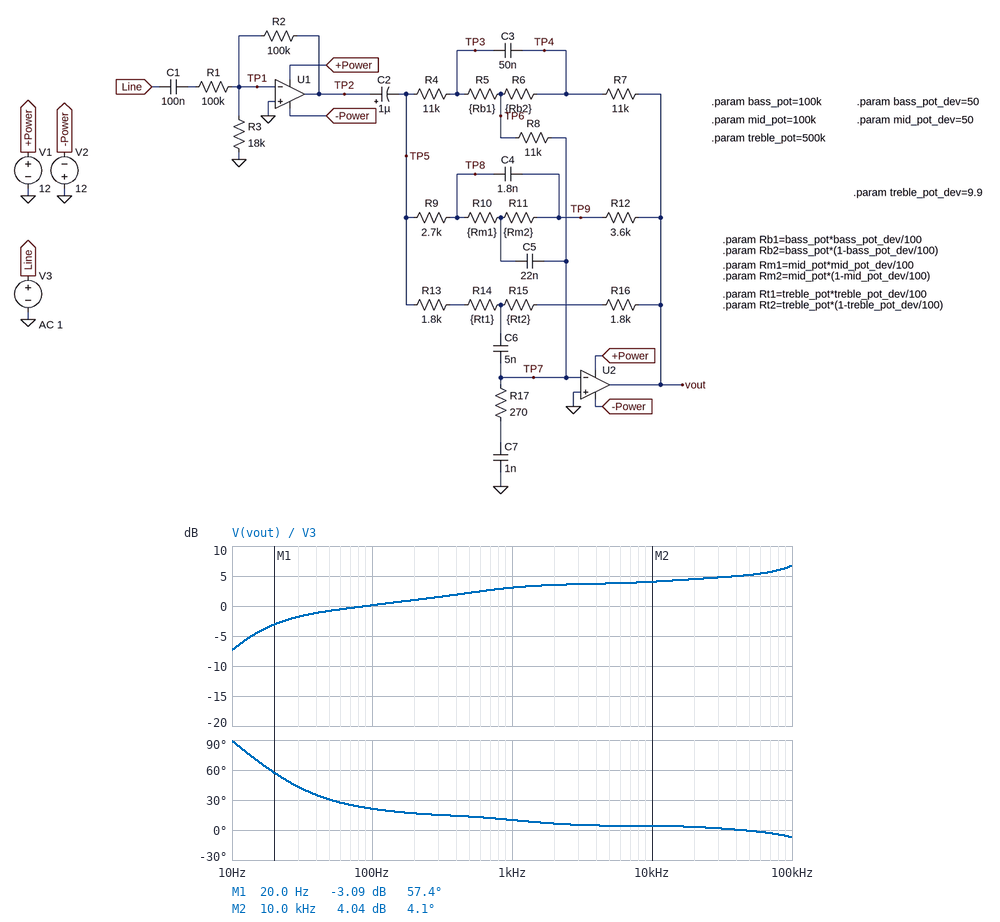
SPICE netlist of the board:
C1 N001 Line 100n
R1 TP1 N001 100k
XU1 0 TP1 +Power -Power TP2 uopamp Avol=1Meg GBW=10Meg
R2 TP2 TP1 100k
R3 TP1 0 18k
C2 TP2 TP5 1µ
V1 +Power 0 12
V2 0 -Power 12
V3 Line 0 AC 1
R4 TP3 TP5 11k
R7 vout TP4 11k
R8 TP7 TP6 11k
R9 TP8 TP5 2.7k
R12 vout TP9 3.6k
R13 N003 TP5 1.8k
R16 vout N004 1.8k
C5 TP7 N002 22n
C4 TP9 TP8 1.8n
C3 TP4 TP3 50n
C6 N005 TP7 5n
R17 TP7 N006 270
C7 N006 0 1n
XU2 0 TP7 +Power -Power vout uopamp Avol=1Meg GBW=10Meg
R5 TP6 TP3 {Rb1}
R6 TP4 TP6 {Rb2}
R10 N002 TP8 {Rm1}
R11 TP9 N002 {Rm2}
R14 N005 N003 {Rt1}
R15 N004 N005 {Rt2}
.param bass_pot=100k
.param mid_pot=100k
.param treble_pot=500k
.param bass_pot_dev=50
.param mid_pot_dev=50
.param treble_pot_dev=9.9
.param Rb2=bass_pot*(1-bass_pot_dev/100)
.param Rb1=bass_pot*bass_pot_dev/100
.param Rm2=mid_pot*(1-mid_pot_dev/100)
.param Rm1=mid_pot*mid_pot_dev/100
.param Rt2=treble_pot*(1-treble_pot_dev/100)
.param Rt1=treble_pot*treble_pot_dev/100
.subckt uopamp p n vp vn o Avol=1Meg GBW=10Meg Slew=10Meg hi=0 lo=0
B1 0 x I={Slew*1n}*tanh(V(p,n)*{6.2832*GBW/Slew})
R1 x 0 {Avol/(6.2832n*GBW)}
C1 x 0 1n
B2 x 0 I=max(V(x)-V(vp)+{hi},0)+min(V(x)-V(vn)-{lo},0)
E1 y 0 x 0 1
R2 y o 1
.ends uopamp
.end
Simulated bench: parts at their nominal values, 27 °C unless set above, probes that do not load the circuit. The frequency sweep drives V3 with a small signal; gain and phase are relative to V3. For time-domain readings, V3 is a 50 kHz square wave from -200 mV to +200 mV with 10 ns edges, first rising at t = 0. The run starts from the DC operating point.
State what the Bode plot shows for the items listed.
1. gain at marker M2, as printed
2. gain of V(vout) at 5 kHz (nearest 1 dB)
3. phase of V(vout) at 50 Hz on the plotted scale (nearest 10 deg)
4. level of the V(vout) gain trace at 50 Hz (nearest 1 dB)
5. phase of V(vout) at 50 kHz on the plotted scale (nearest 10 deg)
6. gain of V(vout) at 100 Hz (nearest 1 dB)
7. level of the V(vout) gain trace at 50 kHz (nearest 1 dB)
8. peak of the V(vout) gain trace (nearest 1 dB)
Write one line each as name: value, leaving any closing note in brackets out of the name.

gain at marker M2, as printed: 4.04 dB
gain of V(vout) at 5 kHz: 4 dB
phase of V(vout) at 50 Hz on the plotted scale: 30 deg
level of the V(vout) gain trace at 50 Hz: -1 dB
phase of V(vout) at 50 kHz on the plotted scale: 0 deg
gain of V(vout) at 100 Hz: 0 dB
level of the V(vout) gain trace at 50 kHz: 5 dB
peak of the V(vout) gain trace: 7 dB
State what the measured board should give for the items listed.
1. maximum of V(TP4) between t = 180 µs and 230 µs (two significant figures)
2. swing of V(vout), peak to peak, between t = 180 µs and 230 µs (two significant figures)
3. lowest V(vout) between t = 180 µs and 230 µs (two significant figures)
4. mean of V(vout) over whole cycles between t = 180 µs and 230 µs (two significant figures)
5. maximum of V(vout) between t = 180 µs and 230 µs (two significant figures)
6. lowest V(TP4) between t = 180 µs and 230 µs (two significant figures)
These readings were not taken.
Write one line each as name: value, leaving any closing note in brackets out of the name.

maximum of V(TP4) between t = 180 µs and 230 µs: 290 mV
swing of V(vout), peak to peak, between t = 180 µs and 230 µs: 1.4 V
lowest V(vout) between t = 180 µs and 230 µs: -470 mV
mean of V(vout) over whole cycles between t = 180 µs and 230 µs: 250 mV
maximum of V(vout) between t = 180 µs and 230 µs: 970 mV
lowest V(TP4) between t = 180 µs and 230 µs: -160 mV
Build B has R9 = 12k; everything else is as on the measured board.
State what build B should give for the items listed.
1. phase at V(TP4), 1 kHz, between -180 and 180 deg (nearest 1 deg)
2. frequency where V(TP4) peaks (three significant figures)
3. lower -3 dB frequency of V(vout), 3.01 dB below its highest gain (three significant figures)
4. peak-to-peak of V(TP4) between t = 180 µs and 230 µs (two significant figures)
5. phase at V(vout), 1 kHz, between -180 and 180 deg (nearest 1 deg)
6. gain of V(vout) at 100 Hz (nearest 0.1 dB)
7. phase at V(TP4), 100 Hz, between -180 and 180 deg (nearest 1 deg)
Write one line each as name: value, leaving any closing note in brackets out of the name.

phase at V(TP4), 1 kHz, between -180 and 180 deg: -32 deg
frequency where V(TP4) peaks: 273 kHz
lower -3 dB frequency of V(vout), 3.01 dB below its highest gain: 168 kHz
peak-to-peak of V(TP4) between t = 180 µs and 230 µs: 280 mV
phase at V(vout), 1 kHz, between -180 and 180 deg: 6 deg
gain of V(vout) at 100 Hz: -0.2 dB
phase at V(TP4), 100 Hz, between -180 and 180 deg: -10 deg
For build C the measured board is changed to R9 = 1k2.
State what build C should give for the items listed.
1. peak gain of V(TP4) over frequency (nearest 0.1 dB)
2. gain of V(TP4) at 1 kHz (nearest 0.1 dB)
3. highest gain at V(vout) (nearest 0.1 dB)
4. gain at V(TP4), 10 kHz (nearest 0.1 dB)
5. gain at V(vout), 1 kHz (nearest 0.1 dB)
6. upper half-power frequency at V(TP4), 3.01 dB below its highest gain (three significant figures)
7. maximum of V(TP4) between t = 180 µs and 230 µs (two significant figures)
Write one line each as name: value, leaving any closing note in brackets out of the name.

peak gain of V(TP4) over frequency: 9.7 dB
gain of V(TP4) at 1 kHz: -12.3 dB
highest gain at V(vout): 17.4 dB
gain at V(TP4), 10 kHz: -9.9 dB
gain at V(vout), 1 kHz: 3.2 dB
upper half-power frequency at V(TP4), 3.01 dB below its highest gain: 229 kHz
maximum of V(TP4) between t = 180 µs and 230 µs: 450 mV
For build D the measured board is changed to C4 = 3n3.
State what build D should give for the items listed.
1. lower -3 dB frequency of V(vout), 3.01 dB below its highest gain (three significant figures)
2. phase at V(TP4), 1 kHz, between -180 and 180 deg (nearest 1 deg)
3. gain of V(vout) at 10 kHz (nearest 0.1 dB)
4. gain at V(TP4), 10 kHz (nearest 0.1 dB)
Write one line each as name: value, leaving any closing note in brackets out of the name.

lower -3 dB frequency of V(vout), 3.01 dB below its highest gain: 155 kHz
phase at V(TP4), 1 kHz, between -180 and 180 deg: -17 deg
gain of V(vout) at 10 kHz: 4.4 dB
gain at V(TP4), 10 kHz: -10.9 dB
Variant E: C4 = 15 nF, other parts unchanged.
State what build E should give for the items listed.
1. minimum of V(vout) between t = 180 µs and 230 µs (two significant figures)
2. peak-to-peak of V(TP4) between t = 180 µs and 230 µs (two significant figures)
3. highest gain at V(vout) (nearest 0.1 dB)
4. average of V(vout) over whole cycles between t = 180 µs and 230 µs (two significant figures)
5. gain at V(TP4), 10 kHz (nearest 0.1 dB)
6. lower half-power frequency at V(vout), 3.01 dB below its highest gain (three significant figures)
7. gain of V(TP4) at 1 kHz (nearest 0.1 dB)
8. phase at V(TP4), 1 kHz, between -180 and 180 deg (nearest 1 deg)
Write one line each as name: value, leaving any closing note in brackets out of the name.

minimum of V(vout) between t = 180 µs and 230 µs: -470 mV
peak-to-peak of V(TP4) between t = 180 µs and 230 µs: 440 mV
highest gain at V(vout): 12.8 dB
average of V(vout) over whole cycles between t = 180 µs and 230 µs: 240 mV
gain at V(TP4), 10 kHz: -9.9 dB
lower half-power frequency at V(vout), 3.01 dB below its highest gain: 155 kHz
gain of V(TP4) at 1 kHz: -12.3 dB
phase at V(TP4), 1 kHz, between -180 and 180 deg: -9 deg
